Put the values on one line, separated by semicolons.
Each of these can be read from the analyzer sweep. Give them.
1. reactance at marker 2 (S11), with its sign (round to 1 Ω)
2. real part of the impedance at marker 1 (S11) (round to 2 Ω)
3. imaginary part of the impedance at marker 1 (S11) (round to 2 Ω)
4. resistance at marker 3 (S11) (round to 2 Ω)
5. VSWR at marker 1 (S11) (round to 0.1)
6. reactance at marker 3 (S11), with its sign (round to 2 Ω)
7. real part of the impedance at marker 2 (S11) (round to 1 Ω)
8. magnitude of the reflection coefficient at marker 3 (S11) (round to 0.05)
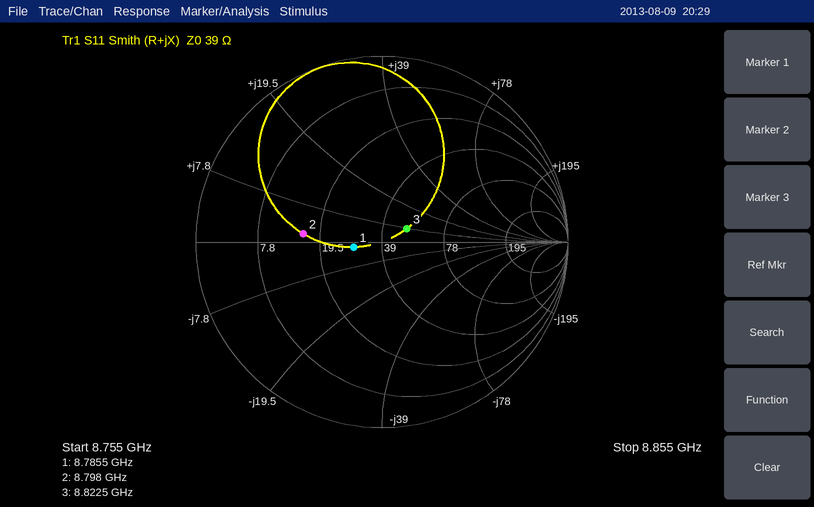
+2 Ω; 28 Ω; -2 Ω; 50 Ω; 1.4; +8 Ω; 16 Ω; 0.15
